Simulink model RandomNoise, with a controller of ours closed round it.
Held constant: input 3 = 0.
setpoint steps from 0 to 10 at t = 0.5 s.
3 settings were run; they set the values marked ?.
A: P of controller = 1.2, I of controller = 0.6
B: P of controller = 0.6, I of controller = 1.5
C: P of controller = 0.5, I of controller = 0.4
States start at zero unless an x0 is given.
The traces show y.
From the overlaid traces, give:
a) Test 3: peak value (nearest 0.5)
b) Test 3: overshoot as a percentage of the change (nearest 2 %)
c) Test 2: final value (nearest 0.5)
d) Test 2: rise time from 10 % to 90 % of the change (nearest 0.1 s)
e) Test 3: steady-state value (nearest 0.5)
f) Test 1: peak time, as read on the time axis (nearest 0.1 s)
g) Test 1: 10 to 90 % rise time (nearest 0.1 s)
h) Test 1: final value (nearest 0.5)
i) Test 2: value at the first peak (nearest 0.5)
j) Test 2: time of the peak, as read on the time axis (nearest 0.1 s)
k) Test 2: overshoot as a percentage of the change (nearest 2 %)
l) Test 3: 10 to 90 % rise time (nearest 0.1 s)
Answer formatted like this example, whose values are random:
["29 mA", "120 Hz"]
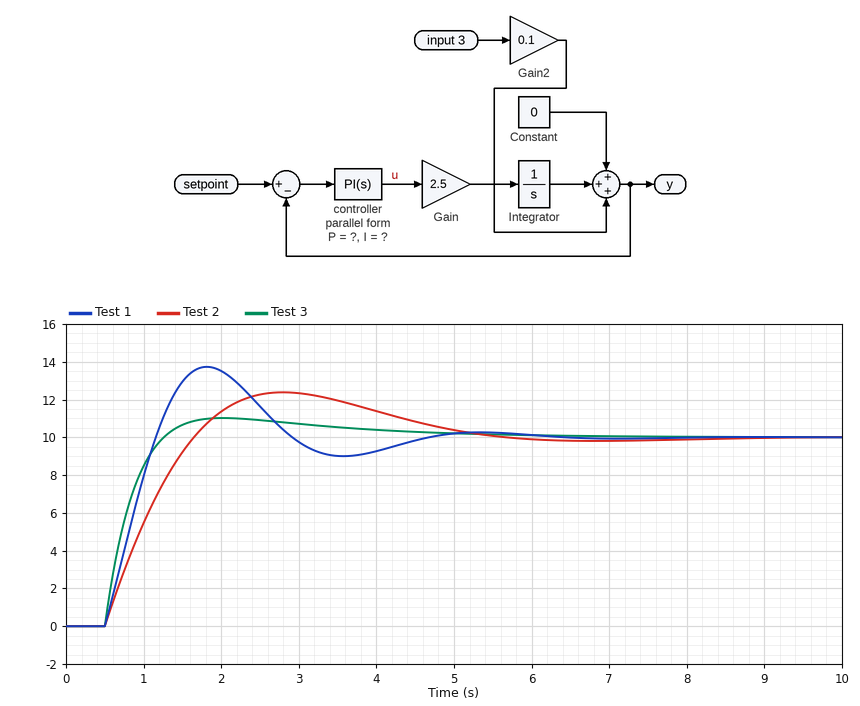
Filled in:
["11.0", "10 %", "10.0", "0.9 s", "10.0", "1.8 s", "0.5 s", "10.0", "12.5", "2.8 s", "24 %", "0.5 s"]
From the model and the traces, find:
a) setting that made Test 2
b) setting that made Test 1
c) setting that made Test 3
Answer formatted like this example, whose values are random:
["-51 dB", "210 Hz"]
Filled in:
["C", "B", "A"]
